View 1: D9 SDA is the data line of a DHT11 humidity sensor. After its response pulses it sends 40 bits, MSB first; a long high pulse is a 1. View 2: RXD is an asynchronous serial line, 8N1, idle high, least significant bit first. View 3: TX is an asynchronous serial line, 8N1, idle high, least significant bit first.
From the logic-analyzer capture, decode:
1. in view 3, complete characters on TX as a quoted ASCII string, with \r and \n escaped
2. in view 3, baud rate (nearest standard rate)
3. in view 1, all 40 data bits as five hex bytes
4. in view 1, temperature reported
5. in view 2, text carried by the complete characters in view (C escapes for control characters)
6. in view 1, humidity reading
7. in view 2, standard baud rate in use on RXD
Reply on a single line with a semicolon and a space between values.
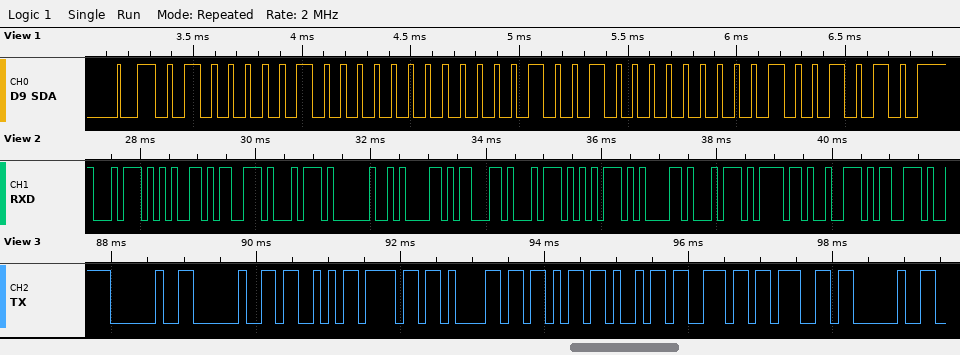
"  Soaking "; 9600 baud; 41 00 09 00 4A; 9.0 °C; "test actuators"; 65 %; 9600 baud
